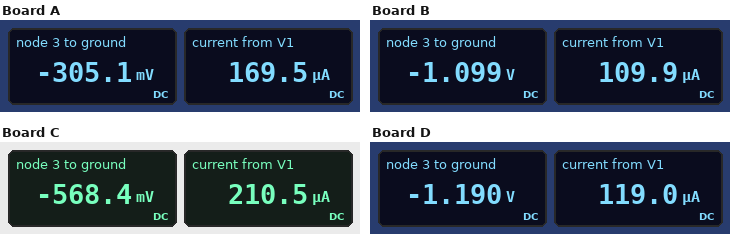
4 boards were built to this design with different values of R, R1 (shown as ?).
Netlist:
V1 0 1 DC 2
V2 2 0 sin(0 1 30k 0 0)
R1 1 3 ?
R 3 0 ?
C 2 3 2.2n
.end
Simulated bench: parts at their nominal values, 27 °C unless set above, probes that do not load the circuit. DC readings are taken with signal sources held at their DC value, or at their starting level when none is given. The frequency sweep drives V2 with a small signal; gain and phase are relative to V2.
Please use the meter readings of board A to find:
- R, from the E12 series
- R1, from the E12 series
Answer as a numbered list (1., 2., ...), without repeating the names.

1. 1.8 kΩ
2. 10 kΩ
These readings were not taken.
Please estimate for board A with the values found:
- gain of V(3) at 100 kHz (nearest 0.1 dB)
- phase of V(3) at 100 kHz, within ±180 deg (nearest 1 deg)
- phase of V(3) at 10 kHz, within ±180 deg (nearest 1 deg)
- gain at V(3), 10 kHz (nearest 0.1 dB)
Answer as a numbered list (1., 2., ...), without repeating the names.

1. -0.9 dB
2. 25 deg
3. 78 deg
4. -13.7 dB
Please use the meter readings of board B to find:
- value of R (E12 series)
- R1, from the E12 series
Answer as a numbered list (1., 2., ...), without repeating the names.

1. 10 kΩ
2. 8.2 kΩ
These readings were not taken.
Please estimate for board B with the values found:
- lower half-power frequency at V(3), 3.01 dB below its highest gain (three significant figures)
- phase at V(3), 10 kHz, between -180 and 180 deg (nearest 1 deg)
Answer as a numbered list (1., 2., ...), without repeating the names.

1. 16.1 kHz
2. 58 deg
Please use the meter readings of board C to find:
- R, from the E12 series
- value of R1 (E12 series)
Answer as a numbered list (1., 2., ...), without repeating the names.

1. 2.7 kΩ
2. 6.8 kΩ
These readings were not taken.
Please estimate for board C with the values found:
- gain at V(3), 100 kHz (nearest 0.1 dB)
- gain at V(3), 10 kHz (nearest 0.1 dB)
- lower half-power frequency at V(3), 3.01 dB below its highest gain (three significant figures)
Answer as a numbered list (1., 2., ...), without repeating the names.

1. -0.6 dB
2. -11.8 dB
3. 37.4 kHz
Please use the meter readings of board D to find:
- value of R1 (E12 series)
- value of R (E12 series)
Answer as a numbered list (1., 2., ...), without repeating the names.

1. 6.8 kΩ
2. 10 kΩ
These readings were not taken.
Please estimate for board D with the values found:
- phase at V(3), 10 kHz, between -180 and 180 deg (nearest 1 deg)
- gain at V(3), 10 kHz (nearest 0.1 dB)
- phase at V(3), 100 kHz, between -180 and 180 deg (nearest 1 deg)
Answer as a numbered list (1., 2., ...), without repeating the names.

1. 61 deg
2. -6.2 dB
3. 10 deg
